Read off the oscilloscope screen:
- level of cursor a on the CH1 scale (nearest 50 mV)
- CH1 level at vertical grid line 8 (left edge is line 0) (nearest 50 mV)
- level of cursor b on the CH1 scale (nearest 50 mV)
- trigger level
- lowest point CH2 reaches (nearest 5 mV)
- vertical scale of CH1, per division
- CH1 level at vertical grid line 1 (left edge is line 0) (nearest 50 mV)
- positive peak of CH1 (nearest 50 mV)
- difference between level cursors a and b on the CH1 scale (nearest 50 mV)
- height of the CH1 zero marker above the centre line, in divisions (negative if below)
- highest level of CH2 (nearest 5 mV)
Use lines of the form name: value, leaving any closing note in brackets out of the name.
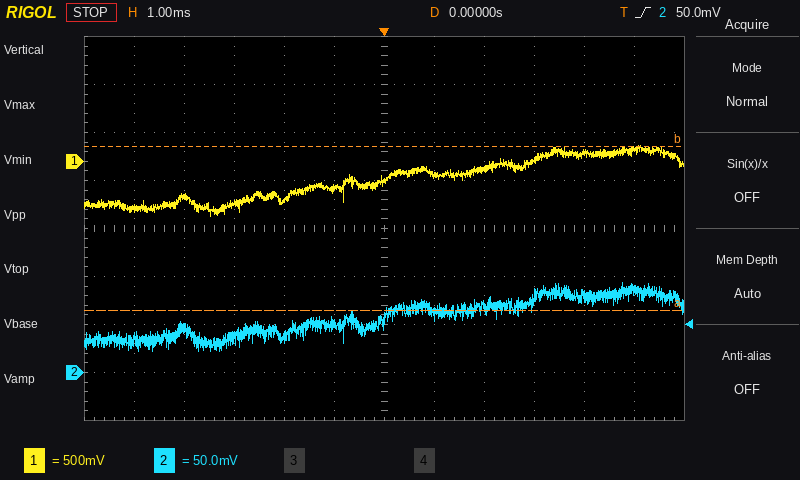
level of cursor a on the CH1 scale: -1.55 V
CH1 level at vertical grid line 8 (left edge is line 0): -100 mV
level of cursor b on the CH1 scale: 150 mV
trigger level: 50.0 mV
lowest point CH2 reaches: 20 mV
vertical scale of CH1, per division: 500 mV
CH1 level at vertical grid line 1 (left edge is line 0): -500 mV
positive peak of CH1: 150 mV
difference between level cursors a and b on the CH1 scale: 1.70 V
height of the CH1 zero marker above the centre line, in divisions: +1.4 div
highest level of CH2: 95 mV
